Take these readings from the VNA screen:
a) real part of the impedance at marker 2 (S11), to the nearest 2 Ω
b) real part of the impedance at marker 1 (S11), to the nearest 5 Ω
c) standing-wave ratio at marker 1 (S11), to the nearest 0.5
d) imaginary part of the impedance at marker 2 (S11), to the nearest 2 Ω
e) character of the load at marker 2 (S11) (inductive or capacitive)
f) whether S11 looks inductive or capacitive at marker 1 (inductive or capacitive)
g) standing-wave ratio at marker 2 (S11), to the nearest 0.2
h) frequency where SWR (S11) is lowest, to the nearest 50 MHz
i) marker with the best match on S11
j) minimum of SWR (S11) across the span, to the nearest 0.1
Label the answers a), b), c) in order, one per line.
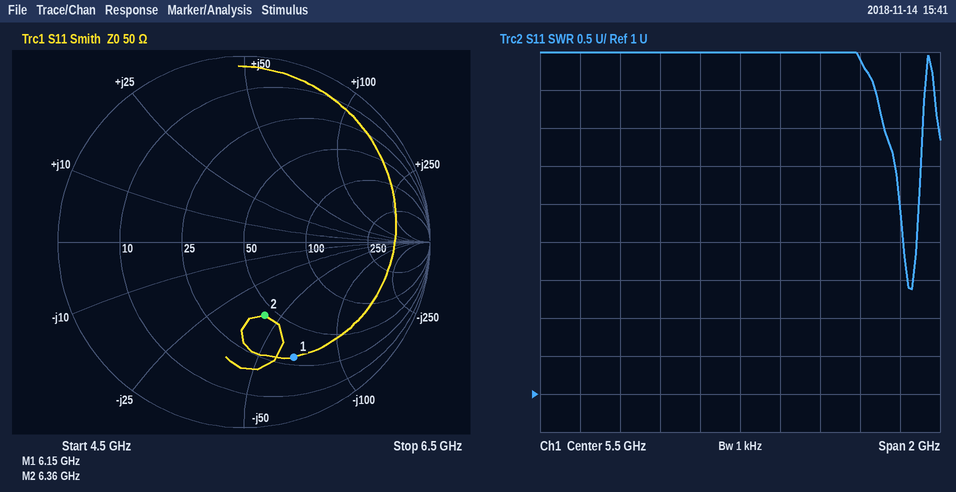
a) 44 Ω
b) 30 Ω
c) 5.0
d) -42 Ω
e) capacitive
f) capacitive
g) 2.4
h) 6.35 GHz
i) marker 2
j) 2.4
